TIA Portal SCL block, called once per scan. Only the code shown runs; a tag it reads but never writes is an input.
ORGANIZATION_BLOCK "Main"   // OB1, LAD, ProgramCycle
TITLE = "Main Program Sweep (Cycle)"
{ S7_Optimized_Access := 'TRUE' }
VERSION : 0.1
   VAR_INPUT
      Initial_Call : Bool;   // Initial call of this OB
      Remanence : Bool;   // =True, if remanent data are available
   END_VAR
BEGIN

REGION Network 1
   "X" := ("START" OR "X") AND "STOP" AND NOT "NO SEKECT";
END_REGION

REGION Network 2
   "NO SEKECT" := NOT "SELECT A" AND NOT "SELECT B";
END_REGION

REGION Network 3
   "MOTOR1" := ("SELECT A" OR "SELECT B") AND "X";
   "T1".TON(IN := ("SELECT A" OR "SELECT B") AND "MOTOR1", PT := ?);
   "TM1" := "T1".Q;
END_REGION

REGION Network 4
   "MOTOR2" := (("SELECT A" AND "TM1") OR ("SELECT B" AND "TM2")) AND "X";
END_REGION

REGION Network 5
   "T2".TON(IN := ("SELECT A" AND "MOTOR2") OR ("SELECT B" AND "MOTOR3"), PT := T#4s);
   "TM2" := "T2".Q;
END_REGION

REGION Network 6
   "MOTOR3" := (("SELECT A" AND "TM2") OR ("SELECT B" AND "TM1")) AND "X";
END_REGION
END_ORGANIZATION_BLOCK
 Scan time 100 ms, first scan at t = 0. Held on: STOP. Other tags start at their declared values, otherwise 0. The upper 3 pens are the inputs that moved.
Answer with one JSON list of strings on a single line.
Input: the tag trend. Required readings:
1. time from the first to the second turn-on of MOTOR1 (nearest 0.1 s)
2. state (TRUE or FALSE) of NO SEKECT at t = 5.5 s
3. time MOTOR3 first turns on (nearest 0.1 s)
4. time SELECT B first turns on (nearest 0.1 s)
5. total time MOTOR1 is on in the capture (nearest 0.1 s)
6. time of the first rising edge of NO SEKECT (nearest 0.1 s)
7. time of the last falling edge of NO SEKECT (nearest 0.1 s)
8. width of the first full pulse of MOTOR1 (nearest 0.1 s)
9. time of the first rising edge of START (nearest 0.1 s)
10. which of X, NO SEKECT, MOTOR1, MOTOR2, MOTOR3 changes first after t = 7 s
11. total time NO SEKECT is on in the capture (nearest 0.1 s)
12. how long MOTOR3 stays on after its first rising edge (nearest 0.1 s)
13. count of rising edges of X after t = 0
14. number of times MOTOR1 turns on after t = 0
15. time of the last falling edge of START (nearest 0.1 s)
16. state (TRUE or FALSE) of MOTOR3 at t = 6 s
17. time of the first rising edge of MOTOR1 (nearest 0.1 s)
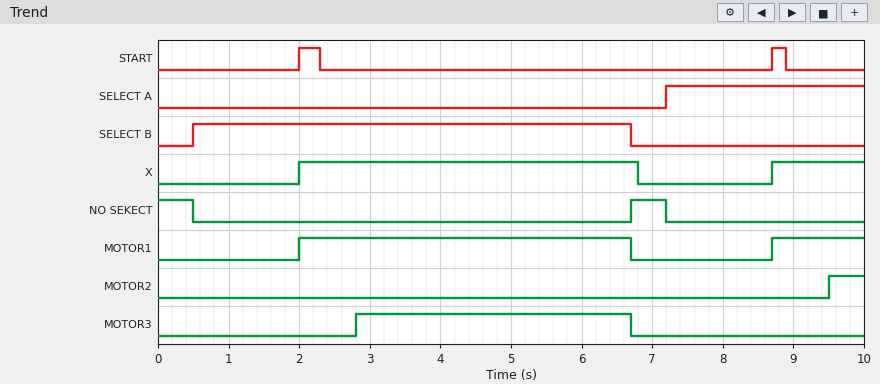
["6.7 s", "FALSE", "2.8 s", "0.5 s", "6.0 s", "6.7 s", "7.2 s", "4.7 s", "2.0 s", "NO SEKECT", "1.0 s", "3.9 s", "2", "2", "8.9 s", "TRUE", "2.0 s"]
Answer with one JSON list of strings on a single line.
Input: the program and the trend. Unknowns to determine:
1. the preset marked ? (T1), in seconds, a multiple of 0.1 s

["0.8 s"]
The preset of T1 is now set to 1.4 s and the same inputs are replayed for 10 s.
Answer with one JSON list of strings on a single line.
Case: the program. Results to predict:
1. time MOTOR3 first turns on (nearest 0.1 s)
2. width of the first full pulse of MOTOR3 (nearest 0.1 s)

["3.4 s", "3.3 s"]
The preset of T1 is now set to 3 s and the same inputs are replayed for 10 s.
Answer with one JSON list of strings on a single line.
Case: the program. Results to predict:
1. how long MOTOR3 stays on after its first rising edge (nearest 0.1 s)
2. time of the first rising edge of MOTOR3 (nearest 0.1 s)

["1.7 s", "5.0 s"]
